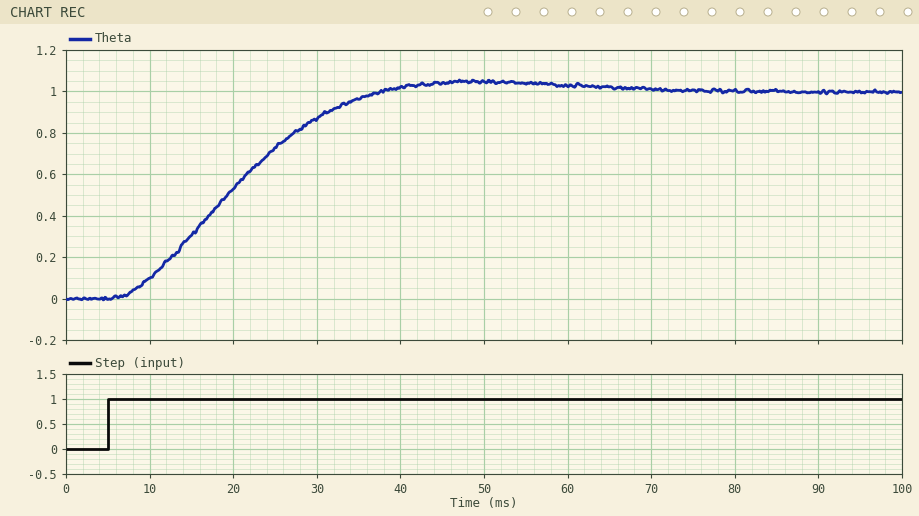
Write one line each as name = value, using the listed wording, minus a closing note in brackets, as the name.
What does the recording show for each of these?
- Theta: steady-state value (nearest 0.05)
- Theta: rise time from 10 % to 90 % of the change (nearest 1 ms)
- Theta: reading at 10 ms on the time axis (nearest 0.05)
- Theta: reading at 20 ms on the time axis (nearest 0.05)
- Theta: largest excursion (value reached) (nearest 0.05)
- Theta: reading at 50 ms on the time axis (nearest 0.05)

Theta: steady-state value = 1.00
Theta: rise time from 10 % to 90 % of the change = 21 ms
Theta: reading at 10 ms on the time axis = 0.10
Theta: reading at 20 ms on the time axis = 0.55
Theta: largest excursion (value reached) = 1.05
Theta: reading at 50 ms on the time axis = 1.05
